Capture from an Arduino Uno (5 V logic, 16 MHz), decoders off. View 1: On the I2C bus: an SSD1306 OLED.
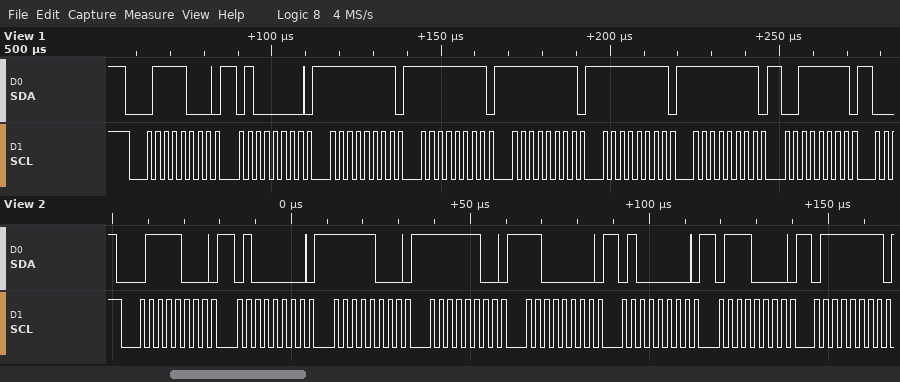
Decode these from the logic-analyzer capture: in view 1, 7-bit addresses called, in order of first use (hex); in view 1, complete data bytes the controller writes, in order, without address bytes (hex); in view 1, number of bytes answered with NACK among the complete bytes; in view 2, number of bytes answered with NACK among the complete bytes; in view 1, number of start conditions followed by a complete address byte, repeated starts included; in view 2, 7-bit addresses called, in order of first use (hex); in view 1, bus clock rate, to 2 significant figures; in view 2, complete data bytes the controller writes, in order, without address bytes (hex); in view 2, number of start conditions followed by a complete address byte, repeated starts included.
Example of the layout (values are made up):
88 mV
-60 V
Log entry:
0x3C
40 FF FF FF FF FF 3F
0
0
1
0x3C
400 kHz
40 F8 FC C0 40 70 7F
1
